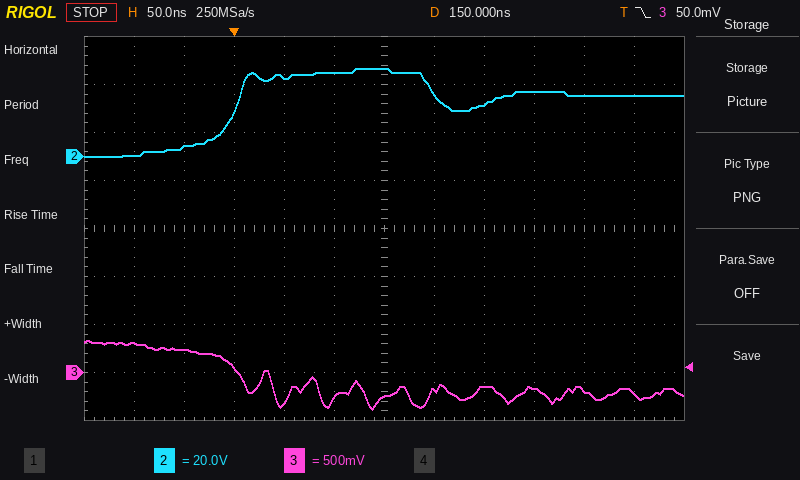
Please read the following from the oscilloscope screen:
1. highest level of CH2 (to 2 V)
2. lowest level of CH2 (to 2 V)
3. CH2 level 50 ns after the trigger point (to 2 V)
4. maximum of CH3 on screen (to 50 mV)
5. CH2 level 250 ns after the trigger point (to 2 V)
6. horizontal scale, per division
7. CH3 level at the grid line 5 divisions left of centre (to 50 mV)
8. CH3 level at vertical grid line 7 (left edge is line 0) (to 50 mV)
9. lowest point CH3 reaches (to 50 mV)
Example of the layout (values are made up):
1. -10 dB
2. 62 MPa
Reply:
1. 36 V
2. 0 V
3. 34 V
4. 350 mV
5. 22 V
6. 50 ns
7. 300 mV
8. -200 mV
9. -400 mV
